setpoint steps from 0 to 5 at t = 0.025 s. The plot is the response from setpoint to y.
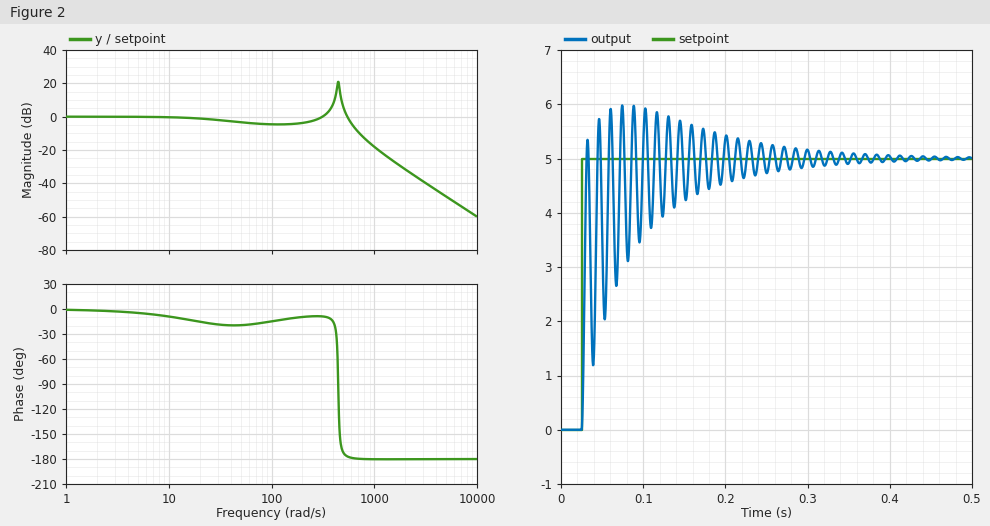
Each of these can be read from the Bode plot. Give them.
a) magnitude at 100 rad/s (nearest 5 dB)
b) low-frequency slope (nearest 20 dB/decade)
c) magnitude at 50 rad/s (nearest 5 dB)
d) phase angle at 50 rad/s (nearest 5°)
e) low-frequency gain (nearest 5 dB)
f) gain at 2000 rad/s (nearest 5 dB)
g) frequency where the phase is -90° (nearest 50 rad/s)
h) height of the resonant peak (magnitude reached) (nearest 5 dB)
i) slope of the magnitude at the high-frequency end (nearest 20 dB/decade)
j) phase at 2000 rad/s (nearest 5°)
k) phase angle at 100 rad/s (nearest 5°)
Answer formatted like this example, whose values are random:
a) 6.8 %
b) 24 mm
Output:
a) -5 dB
b) 0 dB/decade
c) -5 dB
d) -20°
e) 0 dB
f) -30 dB
g) 450 rad/s
h) 20 dB
i) -40 dB/decade
j) -180°
k) -15°
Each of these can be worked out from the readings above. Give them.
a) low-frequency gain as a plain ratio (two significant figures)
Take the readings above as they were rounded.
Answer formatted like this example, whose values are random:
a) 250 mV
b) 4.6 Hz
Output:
a) 1.0
